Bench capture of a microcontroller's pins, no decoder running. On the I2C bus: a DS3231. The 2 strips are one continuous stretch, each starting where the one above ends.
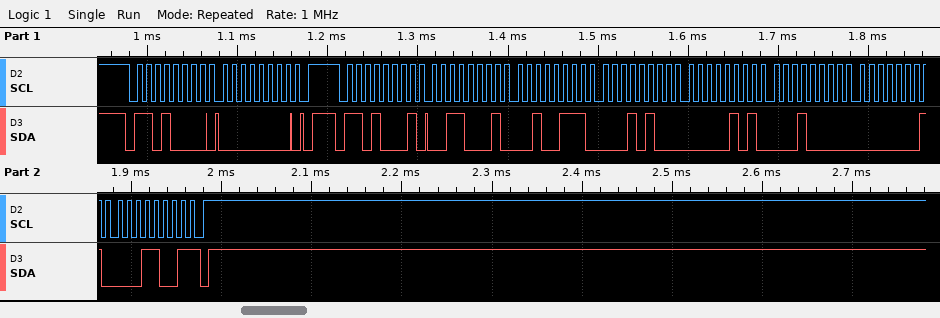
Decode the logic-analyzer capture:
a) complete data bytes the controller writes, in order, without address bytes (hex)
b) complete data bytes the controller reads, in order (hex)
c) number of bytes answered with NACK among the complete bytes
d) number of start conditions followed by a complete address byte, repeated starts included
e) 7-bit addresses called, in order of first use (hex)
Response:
00
31 27 14 05 10 01 19
1
2
0x68
